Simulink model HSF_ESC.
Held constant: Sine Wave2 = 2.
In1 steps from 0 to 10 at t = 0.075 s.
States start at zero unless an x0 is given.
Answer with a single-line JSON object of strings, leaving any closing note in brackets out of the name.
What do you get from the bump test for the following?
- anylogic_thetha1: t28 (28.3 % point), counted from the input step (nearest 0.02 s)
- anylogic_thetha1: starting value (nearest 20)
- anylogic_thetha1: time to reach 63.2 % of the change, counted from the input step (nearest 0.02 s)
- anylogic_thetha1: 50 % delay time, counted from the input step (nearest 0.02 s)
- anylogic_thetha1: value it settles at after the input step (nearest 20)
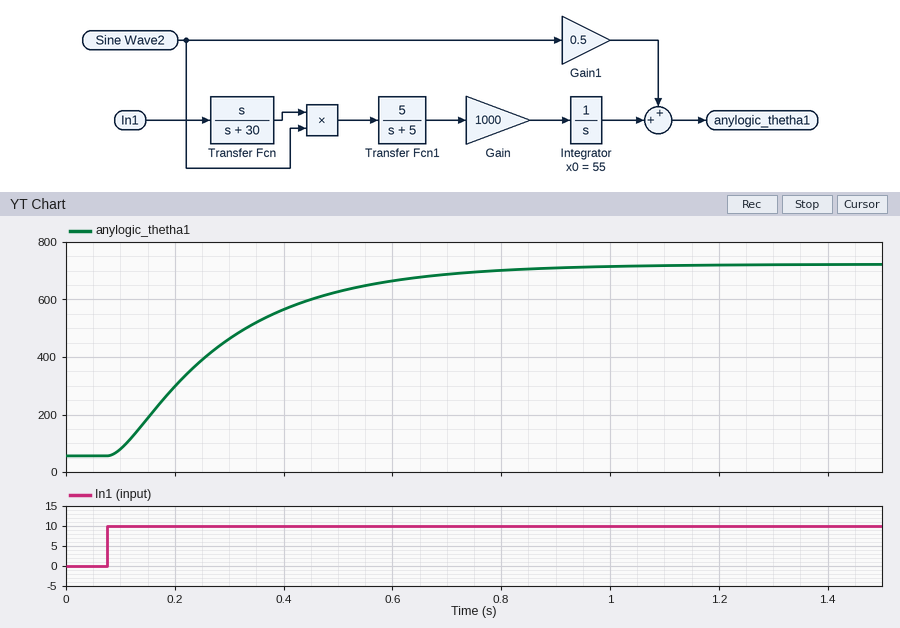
{"anylogic_thetha1: t28 (28.3 % point), counted from the input step": "0.10 s", "anylogic_thetha1: starting value": "60", "anylogic_thetha1: time to reach 63.2 % of the change, counted from the input step": "0.24 s", "anylogic_thetha1: 50 % delay time, counted from the input step": "0.18 s", "anylogic_thetha1: value it settles at after the input step": "720"}
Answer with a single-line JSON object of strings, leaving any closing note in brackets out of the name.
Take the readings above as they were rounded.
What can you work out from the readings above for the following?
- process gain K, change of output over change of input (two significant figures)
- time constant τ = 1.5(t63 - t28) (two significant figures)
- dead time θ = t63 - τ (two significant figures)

{"process gain K, change of output over change of input": "66", "time constant τ = 1.5(t63 - t28)": "0.21 s", "dead time θ = t63 - τ": "0.030 s"}
